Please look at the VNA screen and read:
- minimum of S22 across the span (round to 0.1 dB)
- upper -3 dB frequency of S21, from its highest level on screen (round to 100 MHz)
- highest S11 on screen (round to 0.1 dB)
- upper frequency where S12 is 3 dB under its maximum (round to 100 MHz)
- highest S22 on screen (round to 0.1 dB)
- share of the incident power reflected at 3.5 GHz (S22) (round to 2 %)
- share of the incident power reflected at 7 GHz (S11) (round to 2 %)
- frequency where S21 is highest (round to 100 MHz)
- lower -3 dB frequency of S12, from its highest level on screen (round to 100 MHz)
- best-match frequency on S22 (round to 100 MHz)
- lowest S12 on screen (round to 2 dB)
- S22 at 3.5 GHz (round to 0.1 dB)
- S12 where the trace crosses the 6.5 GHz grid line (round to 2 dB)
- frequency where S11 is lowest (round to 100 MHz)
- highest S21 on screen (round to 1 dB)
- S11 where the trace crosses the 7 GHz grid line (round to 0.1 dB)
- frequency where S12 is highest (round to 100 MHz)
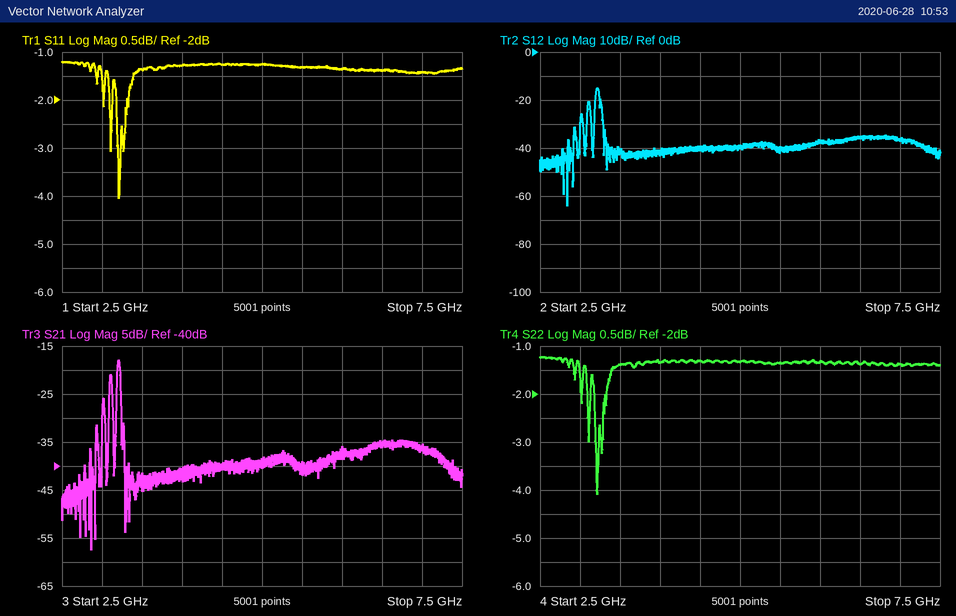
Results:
-4.1 dB
3.2 GHz
-1.2 dB
3.2 GHz
-1.2 dB
72 %
72 %
3.2 GHz
3.2 GHz
3.2 GHz
-64 dB
-1.4 dB
-36 dB
3.2 GHz
-18 dB
-1.4 dB
3.2 GHz
